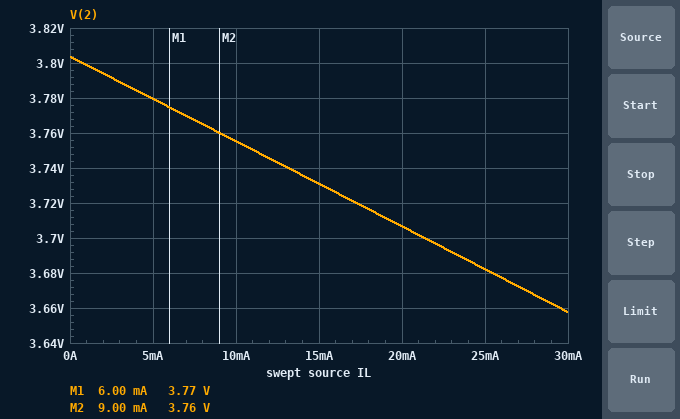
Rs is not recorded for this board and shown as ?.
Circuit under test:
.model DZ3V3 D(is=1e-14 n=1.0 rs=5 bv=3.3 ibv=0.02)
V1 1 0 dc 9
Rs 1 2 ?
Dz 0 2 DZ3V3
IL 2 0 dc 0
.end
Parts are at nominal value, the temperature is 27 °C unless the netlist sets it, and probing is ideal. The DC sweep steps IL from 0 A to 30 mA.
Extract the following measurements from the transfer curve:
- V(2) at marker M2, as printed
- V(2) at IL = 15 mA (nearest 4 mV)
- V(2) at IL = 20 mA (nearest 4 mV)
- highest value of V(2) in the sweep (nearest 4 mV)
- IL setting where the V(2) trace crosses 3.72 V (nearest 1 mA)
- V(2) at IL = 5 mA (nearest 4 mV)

3.76 V
3.732 V
3.708 V
3.804 V
17 mA
3.780 V
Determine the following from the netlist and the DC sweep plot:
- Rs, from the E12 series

56 Ω
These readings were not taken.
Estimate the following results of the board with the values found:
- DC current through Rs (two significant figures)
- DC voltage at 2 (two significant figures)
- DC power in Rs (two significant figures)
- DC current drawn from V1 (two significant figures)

93 mA
3.8 V
480 mW
93 mA
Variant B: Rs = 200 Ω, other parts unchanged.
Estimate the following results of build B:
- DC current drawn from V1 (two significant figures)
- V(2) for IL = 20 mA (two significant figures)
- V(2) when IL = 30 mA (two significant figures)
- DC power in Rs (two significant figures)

28 mA
3.3 V
3.0 V
150 mW
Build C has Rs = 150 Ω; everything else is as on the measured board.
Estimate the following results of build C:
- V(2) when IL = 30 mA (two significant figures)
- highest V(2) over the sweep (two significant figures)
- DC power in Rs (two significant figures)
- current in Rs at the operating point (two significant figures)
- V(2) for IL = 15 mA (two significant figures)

3.3 V
3.5 V
200 mW
37 mA
3.4 V
